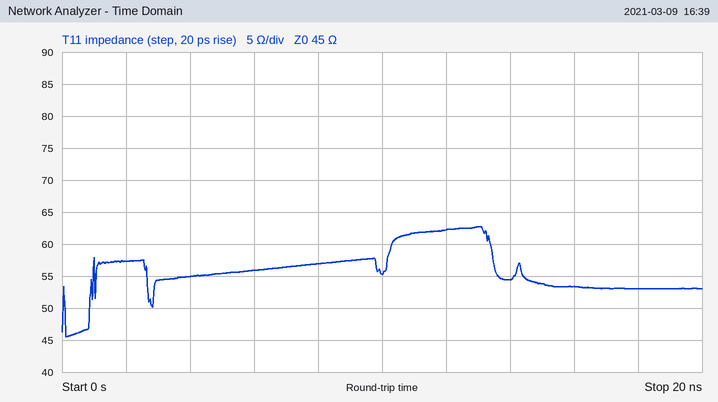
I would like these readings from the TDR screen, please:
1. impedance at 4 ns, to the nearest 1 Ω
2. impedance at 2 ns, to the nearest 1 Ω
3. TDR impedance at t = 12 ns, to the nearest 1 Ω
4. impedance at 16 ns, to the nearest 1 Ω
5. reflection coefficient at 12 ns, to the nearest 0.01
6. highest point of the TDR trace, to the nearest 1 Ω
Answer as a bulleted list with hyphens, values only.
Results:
- 55 Ω
- 57 Ω
- 62 Ω
- 53 Ω
- +0.16
- 63 Ω
